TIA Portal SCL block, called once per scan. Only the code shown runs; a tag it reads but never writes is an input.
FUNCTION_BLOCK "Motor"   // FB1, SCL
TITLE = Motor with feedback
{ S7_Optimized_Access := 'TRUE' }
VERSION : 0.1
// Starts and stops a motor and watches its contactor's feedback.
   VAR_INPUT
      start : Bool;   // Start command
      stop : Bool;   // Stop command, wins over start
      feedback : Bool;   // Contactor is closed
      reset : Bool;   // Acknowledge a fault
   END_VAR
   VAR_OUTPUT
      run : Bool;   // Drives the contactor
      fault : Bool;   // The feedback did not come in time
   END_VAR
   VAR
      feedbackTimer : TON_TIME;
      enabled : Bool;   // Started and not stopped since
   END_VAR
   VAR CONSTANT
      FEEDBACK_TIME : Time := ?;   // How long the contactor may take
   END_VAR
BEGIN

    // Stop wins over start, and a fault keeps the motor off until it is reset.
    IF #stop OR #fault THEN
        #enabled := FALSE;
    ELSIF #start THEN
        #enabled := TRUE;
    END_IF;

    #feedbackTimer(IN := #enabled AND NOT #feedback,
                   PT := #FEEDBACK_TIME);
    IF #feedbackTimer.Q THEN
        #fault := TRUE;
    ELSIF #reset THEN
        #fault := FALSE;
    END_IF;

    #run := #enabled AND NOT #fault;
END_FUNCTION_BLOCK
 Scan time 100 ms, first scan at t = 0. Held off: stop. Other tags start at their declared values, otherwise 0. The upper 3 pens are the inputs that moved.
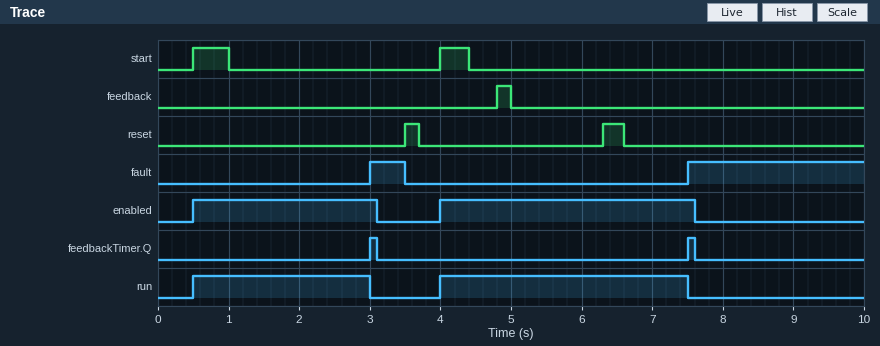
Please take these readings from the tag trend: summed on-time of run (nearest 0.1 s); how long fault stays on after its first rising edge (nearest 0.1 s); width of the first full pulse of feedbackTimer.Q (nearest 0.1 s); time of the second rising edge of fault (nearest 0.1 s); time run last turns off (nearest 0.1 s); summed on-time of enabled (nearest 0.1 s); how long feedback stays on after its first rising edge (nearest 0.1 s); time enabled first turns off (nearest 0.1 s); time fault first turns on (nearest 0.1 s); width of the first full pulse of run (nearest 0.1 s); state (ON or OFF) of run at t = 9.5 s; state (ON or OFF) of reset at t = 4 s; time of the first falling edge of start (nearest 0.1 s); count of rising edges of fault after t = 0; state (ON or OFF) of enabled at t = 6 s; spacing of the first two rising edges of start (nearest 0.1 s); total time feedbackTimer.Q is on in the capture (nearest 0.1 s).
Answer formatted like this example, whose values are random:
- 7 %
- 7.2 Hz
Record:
- 6.0 s
- 0.5 s
- 0.1 s
- 7.5 s
- 7.5 s
- 6.2 s
- 0.2 s
- 3.1 s
- 3.0 s
- 2.5 s
- OFF
- OFF
- 1.0 s
- 2
- ON
- 3.5 s
- 0.2 s
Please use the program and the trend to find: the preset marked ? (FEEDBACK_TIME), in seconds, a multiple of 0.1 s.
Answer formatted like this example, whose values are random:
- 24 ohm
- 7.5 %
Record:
- 2.5 s
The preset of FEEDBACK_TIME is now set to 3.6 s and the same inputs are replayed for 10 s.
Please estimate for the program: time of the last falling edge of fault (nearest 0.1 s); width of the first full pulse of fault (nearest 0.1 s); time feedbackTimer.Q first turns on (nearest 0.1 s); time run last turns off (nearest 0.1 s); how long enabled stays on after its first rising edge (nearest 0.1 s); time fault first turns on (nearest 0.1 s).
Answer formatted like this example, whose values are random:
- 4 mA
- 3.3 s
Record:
- 6.3 s
- 2.2 s
- 4.1 s
- 4.1 s
- 3.7 s
- 4.1 s
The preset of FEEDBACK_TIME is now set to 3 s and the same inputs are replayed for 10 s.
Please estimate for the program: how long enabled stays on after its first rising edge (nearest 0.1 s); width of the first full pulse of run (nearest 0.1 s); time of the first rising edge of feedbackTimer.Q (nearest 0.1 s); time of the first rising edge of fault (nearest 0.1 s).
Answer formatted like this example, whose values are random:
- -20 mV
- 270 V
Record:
- 3.1 s
- 3.0 s
- 3.5 s
- 3.5 s
